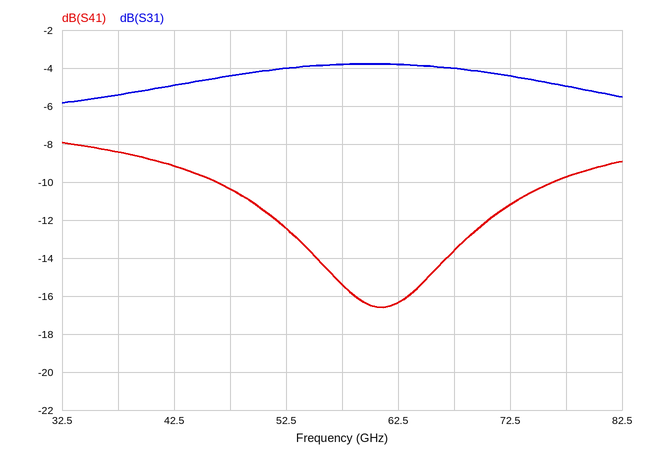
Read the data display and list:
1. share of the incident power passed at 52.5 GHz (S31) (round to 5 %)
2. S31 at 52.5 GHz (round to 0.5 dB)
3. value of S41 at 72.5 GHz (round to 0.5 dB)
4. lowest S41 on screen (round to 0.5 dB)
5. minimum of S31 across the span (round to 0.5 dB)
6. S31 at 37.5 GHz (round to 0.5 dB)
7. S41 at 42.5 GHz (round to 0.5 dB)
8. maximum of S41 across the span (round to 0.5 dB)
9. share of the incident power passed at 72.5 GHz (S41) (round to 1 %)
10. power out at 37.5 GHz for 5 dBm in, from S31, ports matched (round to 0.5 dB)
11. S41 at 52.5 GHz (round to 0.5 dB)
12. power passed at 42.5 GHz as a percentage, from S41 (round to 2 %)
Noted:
40 %
-4.0 dB
-11.0 dB
-16.5 dB
-6.0 dB
-5.5 dB
-9.0 dB
-8.0 dB
8 %
-0.5 dBm
-12.5 dB
12 %
